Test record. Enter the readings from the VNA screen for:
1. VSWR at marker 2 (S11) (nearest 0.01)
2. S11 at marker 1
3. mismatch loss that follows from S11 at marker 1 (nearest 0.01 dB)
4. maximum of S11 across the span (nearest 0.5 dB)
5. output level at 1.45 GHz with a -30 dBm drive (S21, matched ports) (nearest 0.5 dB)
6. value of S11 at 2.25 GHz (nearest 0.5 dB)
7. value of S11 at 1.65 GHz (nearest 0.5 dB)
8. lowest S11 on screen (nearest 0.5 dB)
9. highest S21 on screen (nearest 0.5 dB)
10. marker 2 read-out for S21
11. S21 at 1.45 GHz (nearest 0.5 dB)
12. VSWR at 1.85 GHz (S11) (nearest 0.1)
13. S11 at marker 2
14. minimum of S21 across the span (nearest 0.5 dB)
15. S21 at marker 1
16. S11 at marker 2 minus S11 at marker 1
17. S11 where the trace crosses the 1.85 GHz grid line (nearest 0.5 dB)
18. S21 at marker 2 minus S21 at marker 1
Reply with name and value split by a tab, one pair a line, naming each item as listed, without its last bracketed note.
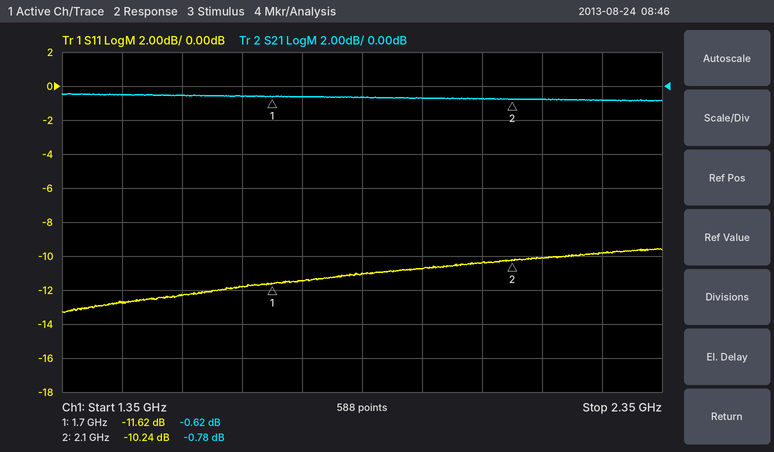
VSWR at marker 2 (S11)	1.89
S11 at marker 1	-11.62 dB
mismatch loss that follows from S11 at marker 1	0.31 dB
maximum of S11 across the span	-9.5 dB
output level at 1.45 GHz with a -30 dBm drive (S21, matched ports)	-30.5 dBm
value of S11 at 2.25 GHz	-10.0 dB
value of S11 at 1.65 GHz	-12.0 dB
lowest S11 on screen	-13.5 dB
highest S21 on screen	-0.5 dB
marker 2 read-out for S21	-0.78 dB
S21 at 1.45 GHz	-0.5 dB
VSWR at 1.85 GHz (S11)	1.8
S11 at marker 2	-10.24 dB
minimum of S21 across the span	-1.0 dB
S21 at marker 1	-0.62 dB
S11 at marker 2 minus S11 at marker 1	1.38 dB
S11 where the trace crosses the 1.85 GHz grid line	-11.0 dB
S21 at marker 2 minus S21 at marker 1	-0.16 dB
